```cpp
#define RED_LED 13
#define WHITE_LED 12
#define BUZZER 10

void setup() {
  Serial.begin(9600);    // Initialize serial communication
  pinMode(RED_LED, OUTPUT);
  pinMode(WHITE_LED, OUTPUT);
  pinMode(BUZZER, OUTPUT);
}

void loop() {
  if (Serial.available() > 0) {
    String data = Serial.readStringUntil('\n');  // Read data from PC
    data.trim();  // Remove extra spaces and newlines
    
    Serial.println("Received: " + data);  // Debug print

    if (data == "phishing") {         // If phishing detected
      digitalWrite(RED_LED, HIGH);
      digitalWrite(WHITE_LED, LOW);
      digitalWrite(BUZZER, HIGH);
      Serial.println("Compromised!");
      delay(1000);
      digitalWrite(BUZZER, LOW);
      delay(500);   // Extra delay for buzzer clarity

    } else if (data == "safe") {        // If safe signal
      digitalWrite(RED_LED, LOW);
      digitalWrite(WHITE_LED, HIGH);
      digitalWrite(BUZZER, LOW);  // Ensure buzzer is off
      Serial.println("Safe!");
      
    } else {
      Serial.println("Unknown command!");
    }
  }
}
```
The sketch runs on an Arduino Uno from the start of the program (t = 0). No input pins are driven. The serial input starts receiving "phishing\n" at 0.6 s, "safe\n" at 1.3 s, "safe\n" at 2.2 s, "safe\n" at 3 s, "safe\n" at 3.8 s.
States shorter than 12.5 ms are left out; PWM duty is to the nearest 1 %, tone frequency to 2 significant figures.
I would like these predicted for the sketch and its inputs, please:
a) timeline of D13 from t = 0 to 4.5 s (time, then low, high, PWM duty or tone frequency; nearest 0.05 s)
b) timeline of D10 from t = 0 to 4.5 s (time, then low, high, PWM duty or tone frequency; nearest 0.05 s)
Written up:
0 s low; 0.6 s high; 2.1 s low
0 s low; 0.6 s high; 1.6 s low
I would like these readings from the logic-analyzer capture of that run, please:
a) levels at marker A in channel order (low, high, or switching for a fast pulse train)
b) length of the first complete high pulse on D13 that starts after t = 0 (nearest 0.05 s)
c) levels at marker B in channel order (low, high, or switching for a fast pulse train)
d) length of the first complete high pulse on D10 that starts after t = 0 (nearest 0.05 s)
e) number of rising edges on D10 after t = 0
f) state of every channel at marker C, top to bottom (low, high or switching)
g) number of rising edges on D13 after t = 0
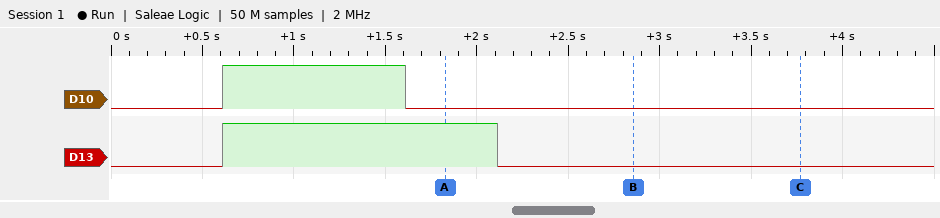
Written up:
D10 low, D13 high
1.50 s
D10 low, D13 low
1.00 s
1
D10 low, D13 low
1
